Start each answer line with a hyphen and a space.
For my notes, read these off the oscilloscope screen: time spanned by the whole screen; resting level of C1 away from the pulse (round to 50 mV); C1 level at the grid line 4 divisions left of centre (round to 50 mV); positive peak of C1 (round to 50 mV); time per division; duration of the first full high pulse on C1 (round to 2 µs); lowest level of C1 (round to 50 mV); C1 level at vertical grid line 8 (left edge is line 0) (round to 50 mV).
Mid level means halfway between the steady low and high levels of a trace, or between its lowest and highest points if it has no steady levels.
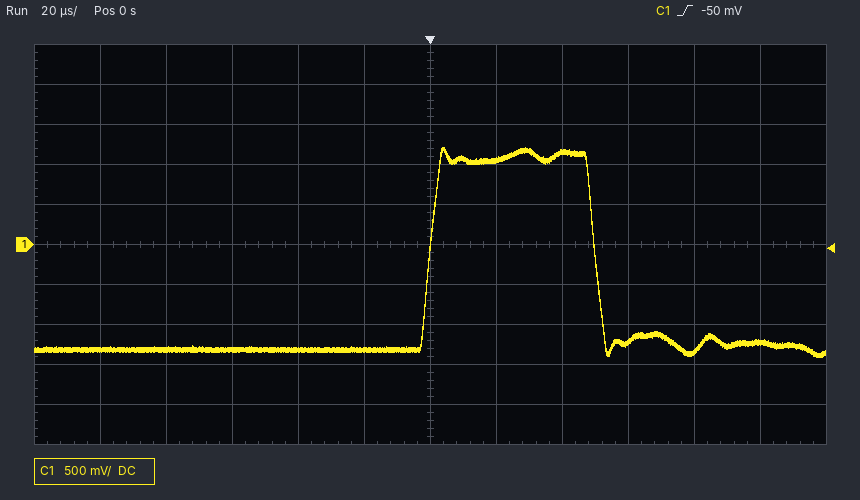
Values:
- 240 µs
- -1.30 V
- -1.30 V
- 1.20 V
- 20 µs
- 50 µs
- -1.40 V
- 1.15 V
